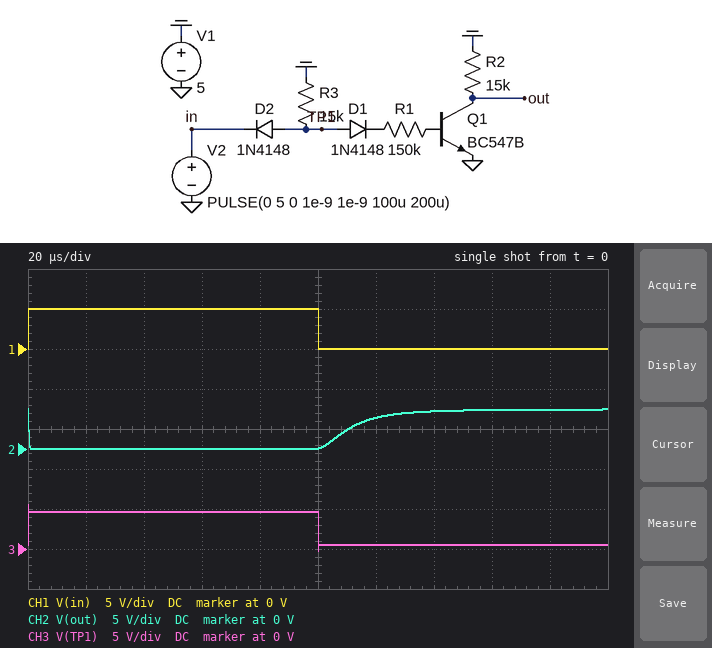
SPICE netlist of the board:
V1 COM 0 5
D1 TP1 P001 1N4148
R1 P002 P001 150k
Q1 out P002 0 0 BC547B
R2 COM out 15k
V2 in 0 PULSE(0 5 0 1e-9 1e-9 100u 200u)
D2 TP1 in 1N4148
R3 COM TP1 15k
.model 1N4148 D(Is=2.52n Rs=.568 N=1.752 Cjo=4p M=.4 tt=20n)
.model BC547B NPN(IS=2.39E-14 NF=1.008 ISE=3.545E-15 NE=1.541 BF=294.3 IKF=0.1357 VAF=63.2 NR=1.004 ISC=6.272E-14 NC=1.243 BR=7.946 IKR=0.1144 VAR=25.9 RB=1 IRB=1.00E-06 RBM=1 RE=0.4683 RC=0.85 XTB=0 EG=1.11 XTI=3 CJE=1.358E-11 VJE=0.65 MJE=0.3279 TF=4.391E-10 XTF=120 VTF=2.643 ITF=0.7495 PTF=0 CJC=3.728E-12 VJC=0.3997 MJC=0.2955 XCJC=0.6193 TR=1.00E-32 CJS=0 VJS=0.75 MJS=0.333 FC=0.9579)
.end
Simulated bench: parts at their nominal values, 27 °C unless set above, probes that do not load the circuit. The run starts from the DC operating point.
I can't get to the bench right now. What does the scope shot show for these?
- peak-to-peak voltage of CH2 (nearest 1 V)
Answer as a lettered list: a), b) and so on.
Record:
a) 5 V
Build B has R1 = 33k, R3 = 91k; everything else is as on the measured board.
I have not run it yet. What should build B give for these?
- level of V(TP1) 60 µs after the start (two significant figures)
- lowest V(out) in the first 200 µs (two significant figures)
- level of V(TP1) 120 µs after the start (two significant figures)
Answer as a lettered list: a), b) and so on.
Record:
a) 2.1 V
b) 29 mV
c) 450 mV
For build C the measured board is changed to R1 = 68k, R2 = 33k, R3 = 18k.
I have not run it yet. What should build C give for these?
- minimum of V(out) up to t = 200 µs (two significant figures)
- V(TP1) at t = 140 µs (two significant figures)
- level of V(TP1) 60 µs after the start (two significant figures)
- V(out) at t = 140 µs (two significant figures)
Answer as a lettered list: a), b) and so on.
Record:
a) 15 mV
b) 520 mV
c) 4.2 V
d) 3.8 V
